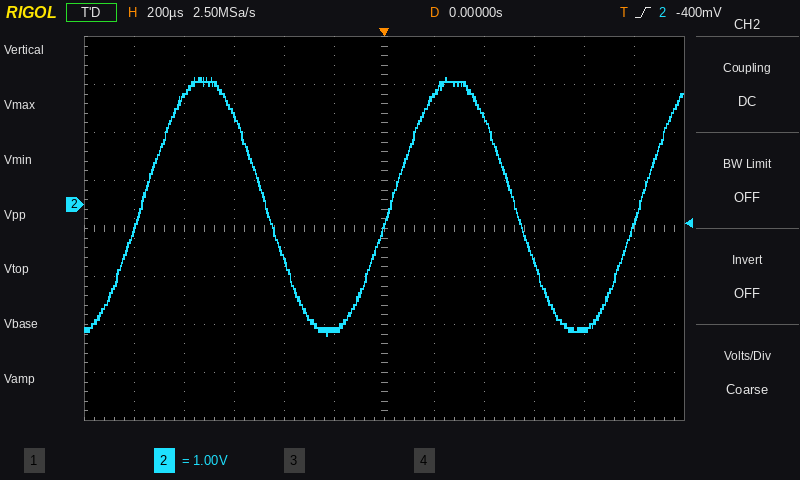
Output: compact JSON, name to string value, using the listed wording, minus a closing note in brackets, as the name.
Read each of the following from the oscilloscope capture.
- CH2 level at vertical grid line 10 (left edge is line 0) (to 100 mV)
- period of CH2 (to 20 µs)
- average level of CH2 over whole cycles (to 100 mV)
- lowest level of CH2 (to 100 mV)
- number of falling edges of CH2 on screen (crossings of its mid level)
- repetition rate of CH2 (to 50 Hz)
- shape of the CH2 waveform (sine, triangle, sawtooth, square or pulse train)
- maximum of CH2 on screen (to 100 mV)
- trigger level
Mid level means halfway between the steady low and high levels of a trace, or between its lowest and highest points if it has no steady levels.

{"CH2 level at vertical grid line 10 (left edge is line 0)": "-2.6 V", "period of CH2": "1.00 ms", "average level of CH2 over whole cycles": "0.0 V", "lowest level of CH2": "-2.7 V", "number of falling edges of CH2 on screen": "2", "repetition rate of CH2": "1.00 kHz", "shape of the CH2 waveform": "sine", "maximum of CH2 on screen": "2.6 V", "trigger level": "-400 mV"}
